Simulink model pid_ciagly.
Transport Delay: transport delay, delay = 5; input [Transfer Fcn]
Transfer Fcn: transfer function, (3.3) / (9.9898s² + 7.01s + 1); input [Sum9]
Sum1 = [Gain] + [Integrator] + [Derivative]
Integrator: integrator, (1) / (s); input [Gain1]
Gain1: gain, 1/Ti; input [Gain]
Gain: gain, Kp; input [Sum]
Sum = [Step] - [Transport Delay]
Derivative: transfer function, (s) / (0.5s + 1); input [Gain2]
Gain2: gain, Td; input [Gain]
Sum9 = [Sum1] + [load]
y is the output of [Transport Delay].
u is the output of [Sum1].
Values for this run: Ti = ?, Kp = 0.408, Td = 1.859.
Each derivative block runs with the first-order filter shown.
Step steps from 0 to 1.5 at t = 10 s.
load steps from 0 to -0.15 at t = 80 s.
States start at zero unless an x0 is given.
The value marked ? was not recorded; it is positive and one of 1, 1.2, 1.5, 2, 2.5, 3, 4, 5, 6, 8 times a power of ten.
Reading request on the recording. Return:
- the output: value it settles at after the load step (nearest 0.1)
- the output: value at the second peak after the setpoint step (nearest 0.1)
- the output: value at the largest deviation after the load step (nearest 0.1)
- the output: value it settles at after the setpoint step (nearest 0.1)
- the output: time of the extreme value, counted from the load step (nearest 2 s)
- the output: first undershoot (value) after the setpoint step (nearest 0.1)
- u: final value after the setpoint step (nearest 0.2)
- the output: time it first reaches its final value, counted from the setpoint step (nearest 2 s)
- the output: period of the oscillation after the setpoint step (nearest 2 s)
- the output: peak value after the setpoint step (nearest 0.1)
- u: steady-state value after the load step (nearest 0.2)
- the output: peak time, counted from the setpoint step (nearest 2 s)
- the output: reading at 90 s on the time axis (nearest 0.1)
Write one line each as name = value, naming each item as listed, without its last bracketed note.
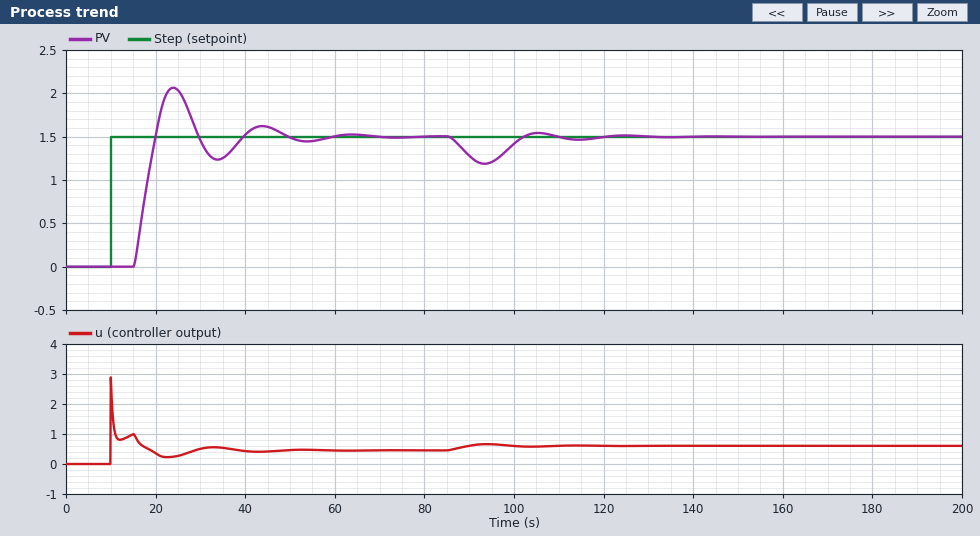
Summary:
the output: value it settles at after the load step = 1.5
the output: value at the second peak after the setpoint step = 1.6
the output: value at the largest deviation after the load step = 1.2
the output: value it settles at after the setpoint step = 1.5
the output: time of the extreme value, counted from the load step = 14 s
the output: first undershoot (value) after the setpoint step = 1.2
u: final value after the setpoint step = 0.4
the output: time it first reaches its final value, counted from the setpoint step = 10 s
the output: period of the oscillation after the setpoint step = 20 s
the output: peak value after the setpoint step = 2.1
u: steady-state value after the load step = 0.6
the output: peak time, counted from the setpoint step = 14 s
the output: reading at 90 s on the time axis = 1.3
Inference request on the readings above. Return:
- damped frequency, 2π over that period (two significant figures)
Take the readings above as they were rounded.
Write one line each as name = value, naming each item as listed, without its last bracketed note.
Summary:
damped frequency, 2π over that period = 0.31 rad/s
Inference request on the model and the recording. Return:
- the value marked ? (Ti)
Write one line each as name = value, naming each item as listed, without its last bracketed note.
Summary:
the value marked ? = 8
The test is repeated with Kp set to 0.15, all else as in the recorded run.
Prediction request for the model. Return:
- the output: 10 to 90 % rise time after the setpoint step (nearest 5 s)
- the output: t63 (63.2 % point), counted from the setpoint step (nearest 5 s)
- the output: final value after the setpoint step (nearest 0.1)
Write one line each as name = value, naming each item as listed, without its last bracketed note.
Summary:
the output: 10 to 90 % rise time after the setpoint step = 25 s
the output: t63 (63.2 % point), counted from the setpoint step = 15 s
the output: final value after the setpoint step = 1.5
